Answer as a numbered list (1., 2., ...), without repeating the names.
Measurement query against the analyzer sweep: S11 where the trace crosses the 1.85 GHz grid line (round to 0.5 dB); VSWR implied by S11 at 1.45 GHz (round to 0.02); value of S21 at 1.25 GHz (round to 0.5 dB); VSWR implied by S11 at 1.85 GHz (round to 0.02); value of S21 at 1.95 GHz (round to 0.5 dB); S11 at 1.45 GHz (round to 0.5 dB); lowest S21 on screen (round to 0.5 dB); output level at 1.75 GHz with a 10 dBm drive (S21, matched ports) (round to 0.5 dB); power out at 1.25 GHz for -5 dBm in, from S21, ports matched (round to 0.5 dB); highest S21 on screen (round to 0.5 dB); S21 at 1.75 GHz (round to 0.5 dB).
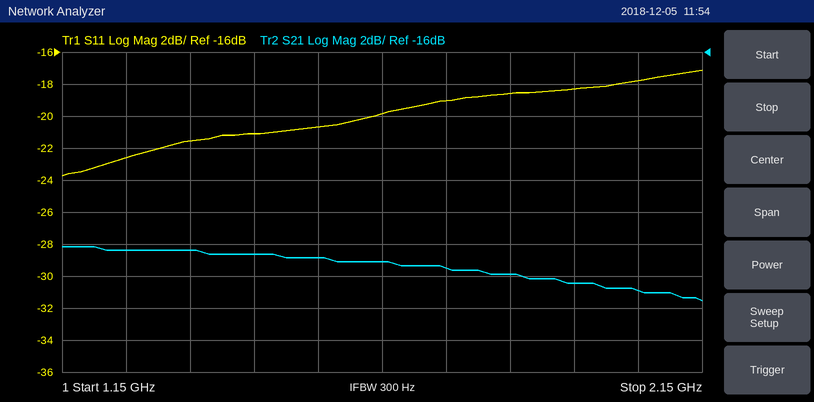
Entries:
1. -18.5 dB
2. 1.20
3. -28.5 dB
4. 1.26
5. -30.5 dB
6. -21.0 dB
7. -31.5 dB
8. -19.5 dBm
9. -33.5 dBm
10. -28.0 dB
11. -29.5 dB
